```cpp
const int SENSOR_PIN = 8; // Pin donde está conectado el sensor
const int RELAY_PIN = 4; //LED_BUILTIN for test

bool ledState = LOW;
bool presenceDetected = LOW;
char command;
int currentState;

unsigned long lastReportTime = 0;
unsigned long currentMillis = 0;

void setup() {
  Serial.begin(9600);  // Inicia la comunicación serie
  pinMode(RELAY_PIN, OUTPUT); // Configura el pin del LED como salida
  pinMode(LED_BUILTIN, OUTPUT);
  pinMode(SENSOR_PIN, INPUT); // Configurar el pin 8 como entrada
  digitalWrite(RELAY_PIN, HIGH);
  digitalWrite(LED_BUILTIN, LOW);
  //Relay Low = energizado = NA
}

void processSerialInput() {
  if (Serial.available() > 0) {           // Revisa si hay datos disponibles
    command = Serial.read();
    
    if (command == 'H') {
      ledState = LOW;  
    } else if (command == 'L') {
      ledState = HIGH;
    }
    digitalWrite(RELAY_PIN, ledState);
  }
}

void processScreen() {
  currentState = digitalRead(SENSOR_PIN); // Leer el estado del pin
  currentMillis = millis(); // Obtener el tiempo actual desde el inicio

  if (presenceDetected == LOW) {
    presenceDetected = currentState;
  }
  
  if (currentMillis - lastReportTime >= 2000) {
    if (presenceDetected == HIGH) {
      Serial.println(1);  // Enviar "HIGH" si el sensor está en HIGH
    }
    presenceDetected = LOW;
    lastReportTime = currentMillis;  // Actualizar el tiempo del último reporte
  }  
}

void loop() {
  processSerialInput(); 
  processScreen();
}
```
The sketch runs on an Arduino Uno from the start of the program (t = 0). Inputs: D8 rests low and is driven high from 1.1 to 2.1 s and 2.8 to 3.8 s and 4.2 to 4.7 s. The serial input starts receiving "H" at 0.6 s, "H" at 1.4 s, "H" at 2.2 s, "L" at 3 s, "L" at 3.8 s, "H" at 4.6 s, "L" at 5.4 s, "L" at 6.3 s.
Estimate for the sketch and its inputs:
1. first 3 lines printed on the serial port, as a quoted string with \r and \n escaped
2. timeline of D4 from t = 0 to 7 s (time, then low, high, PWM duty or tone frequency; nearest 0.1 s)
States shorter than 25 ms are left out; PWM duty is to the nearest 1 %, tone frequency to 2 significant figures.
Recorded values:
"1\r\n1\r\n1\r\n"
0 s high; 0.6 s low; 3 s high; 4.6 s low; 5.4 s high
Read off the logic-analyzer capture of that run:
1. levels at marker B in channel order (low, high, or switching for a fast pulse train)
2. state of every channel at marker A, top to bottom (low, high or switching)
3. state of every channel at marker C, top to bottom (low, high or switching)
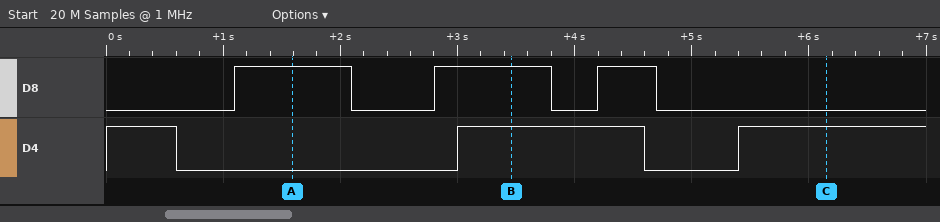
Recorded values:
D8 high, D4 high
D8 high, D4 low
D8 low, D4 high
